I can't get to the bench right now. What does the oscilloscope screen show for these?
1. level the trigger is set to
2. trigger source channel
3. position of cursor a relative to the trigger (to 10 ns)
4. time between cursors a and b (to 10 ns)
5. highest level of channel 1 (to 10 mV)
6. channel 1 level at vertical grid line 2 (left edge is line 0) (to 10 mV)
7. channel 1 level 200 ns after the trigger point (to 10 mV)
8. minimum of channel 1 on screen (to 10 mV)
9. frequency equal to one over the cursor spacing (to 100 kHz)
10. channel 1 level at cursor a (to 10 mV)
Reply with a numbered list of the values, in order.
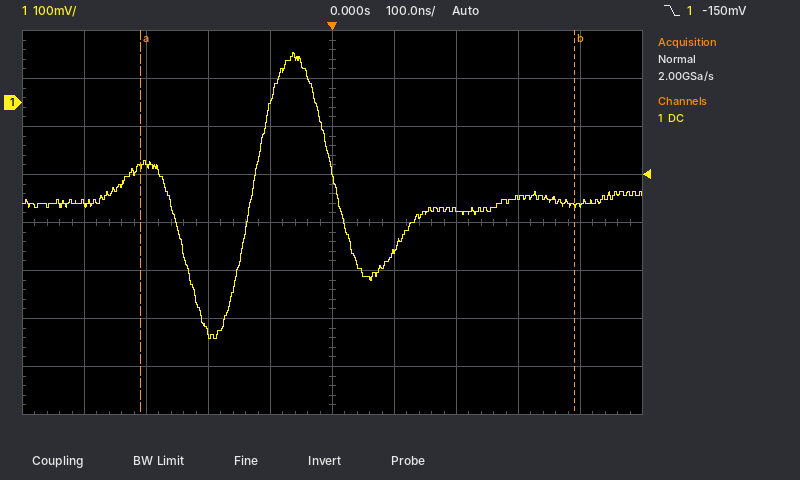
1. -150 mV
2. channel 1
3. -310 ns
4. 700 ns
5. 100 mV
6. -130 mV
7. -220 mV
8. -490 mV
9. 1.4 MHz
10. -130 mV
